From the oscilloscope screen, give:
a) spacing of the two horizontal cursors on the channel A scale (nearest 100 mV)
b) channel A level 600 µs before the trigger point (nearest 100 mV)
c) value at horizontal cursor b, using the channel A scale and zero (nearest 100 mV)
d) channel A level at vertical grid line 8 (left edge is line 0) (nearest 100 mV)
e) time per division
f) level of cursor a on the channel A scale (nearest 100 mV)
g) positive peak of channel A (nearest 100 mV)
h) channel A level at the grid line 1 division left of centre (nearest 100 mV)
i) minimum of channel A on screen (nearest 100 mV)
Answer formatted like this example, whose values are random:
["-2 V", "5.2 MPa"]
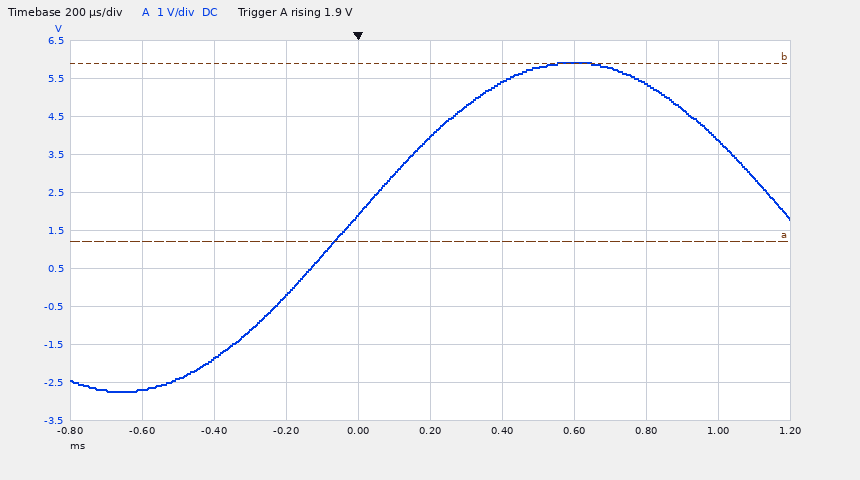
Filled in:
["4.7 V", "-2.7 V", "5.9 V", "5.4 V", "200 µs", "1.2 V", "5.9 V", "1.9 V", "-2.7 V"]
